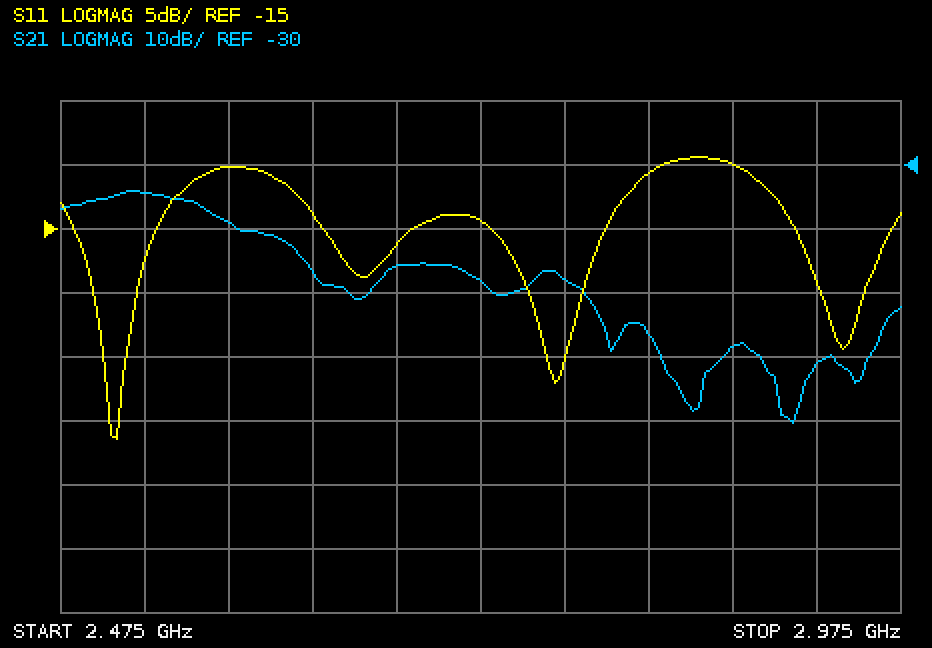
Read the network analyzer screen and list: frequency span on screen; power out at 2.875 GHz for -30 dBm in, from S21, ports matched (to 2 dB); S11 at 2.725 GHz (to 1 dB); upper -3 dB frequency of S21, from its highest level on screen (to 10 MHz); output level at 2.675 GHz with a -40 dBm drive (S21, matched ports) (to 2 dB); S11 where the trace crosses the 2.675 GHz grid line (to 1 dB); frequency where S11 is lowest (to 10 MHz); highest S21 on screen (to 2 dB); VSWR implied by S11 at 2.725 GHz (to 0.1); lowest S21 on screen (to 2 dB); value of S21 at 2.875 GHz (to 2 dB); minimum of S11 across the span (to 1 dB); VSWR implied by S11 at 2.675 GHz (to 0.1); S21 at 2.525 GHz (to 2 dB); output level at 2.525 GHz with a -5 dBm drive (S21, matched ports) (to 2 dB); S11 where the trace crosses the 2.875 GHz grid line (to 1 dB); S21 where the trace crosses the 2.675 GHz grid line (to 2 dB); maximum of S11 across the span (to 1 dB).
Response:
500 MHz
-88 dBm
-14 dB
2.56 GHz
-86 dBm
-16 dB
2.51 GHz
-34 dB
1.5
-70 dB
-58 dB
-31 dB
1.4
-34 dB
-40 dBm
-10 dB
-46 dB
-9 dB
